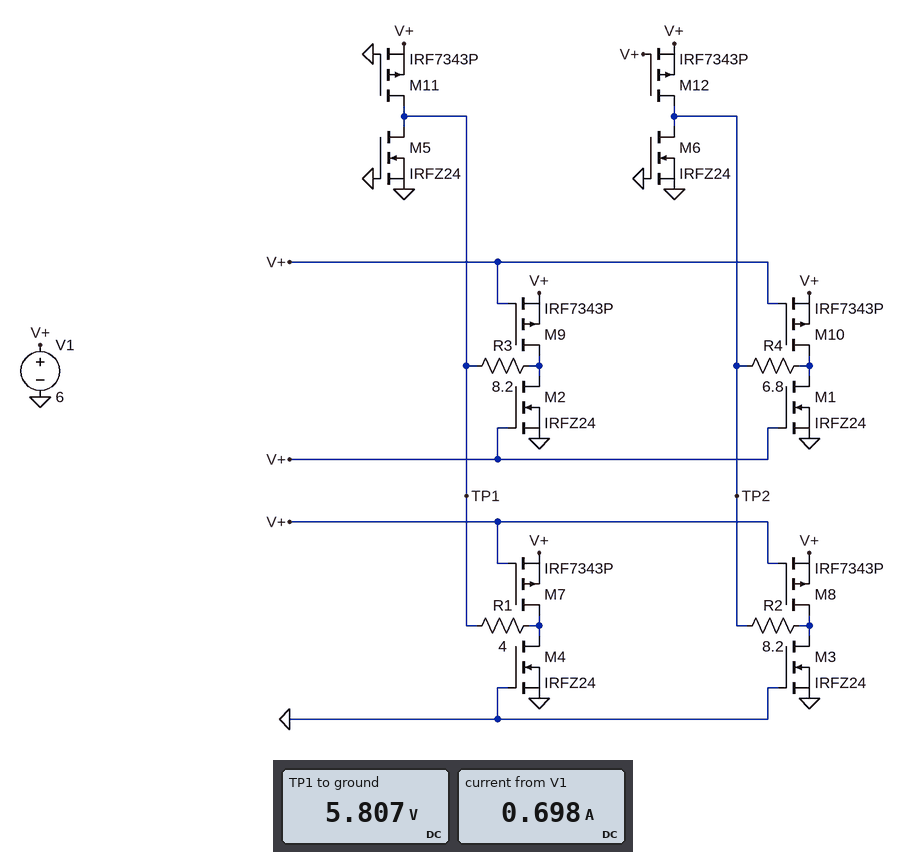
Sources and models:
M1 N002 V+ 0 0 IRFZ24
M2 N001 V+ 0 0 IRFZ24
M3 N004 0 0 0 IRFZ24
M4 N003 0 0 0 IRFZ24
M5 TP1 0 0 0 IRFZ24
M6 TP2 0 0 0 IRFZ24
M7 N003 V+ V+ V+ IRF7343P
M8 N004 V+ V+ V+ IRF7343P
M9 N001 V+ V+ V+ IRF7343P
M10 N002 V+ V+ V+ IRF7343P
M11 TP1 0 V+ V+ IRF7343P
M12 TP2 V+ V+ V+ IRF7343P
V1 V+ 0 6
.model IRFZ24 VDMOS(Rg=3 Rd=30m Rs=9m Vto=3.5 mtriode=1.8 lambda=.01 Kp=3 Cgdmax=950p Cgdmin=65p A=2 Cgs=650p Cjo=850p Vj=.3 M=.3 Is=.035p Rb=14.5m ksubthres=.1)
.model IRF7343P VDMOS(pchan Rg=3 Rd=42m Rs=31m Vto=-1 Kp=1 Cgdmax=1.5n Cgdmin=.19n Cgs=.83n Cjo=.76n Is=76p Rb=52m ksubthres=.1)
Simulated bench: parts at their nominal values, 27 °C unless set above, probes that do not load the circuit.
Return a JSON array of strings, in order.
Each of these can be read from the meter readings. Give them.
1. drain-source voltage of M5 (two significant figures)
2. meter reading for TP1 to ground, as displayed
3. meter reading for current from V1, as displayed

["5.8 V", "5.807 V", "0.698 A"]
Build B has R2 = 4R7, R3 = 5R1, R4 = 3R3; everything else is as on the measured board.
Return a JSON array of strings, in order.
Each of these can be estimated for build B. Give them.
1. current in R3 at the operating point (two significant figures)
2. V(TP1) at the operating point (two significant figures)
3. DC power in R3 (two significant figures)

["1.1 A", "5.7 V", "6.1 W"]
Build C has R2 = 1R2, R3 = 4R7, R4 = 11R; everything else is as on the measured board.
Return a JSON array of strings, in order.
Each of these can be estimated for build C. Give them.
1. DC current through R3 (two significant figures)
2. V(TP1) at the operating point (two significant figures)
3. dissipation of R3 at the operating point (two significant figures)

["1.2 A", "5.7 V", "6.5 W"]
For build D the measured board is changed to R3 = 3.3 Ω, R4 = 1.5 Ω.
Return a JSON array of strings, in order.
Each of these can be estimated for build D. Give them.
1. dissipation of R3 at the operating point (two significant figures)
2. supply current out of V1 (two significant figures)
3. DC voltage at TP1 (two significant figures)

["8.7 W", "1.6 A", "5.5 V"]
